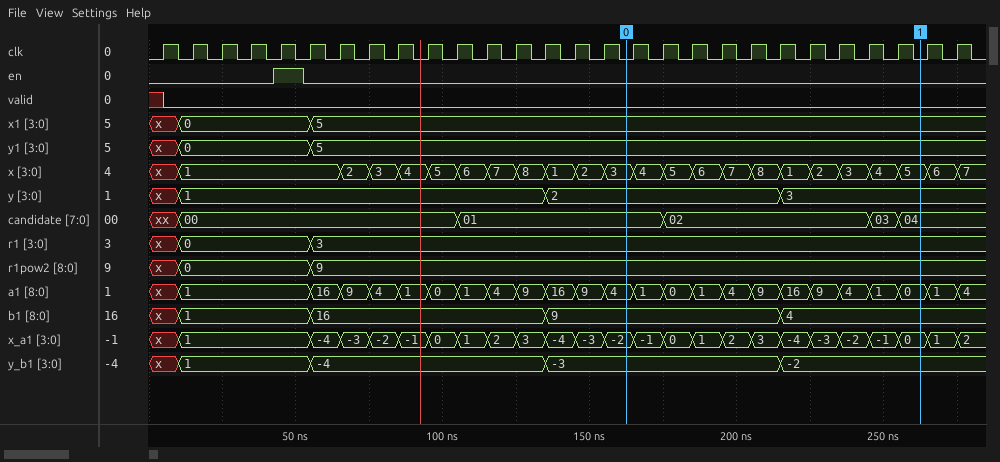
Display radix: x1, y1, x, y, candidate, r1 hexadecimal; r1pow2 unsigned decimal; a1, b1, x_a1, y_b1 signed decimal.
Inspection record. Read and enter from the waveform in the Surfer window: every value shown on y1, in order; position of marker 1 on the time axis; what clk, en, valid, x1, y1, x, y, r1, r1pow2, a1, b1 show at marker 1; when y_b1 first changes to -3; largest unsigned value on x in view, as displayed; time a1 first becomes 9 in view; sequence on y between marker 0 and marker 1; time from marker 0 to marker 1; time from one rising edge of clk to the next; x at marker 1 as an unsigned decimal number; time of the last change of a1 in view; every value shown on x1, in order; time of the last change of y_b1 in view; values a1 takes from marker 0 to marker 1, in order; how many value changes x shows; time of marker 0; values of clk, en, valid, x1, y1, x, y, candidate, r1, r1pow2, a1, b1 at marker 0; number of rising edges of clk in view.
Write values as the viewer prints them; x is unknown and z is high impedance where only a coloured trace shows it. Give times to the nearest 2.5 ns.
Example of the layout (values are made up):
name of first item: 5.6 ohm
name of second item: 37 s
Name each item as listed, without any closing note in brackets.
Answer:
every value shown on y1, in order: x, 0, 5
position of marker 1 on the time axis: 262.5 ns
what clk, en, valid, x1, y1, x, y, r1, r1pow2, a1, b1 show at marker 1: clk=0, en=0, valid=0, x1=5, y1=5, x=5, y=3, r1=3, r1pow2=9, a1=0, b1=4
when y_b1 first changes to -3: 135 ns
largest unsigned value on x in view, as displayed: 8
time a1 first becomes 9 in view: 65 ns
sequence on y between marker 0 and marker 1: 2, 3
time from marker 0 to marker 1: 100 ns
time from one rising edge of clk to the next: 10 ns
x at marker 1 as an unsigned decimal number: 5
time of the last change of a1 in view: 275 ns
every value shown on x1, in order: x, 0, 5
time of the last change of y_b1 in view: 215 ns
values a1 takes from marker 0 to marker 1, in order: 4, 1, 0, 1, 4, 9, 16, 9, 4, 1, 0
how many value changes x shows: 23
time of marker 0: 162.5 ns
values of clk, en, valid, x1, y1, x, y, candidate, r1, r1pow2, a1, b1 at marker 0: clk=0, en=0, valid=0, x1=5, y1=5, x=3, y=2, candidate=01, r1=3, r1pow2=9, a1=4, b1=9
number of rising edges of clk in view: 28
